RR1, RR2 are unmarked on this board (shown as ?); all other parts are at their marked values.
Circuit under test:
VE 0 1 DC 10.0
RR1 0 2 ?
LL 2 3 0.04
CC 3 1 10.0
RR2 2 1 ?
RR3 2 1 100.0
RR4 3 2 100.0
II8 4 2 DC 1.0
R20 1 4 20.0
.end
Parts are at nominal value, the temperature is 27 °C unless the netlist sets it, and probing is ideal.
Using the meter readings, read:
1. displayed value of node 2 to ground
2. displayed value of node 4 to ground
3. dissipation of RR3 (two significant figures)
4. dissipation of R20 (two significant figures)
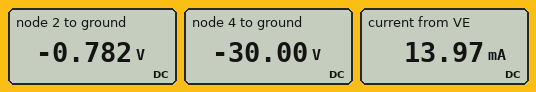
-0.782 V
-30.00 V
850 mW
20 W
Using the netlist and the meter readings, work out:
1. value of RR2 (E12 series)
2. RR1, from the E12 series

10 Ω
56 Ω
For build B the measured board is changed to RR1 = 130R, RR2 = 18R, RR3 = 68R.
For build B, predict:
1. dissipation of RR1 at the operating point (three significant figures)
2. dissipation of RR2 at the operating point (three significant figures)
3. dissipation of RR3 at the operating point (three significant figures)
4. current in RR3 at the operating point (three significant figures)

112 mW
10.6 W
2.81 W
203 mA
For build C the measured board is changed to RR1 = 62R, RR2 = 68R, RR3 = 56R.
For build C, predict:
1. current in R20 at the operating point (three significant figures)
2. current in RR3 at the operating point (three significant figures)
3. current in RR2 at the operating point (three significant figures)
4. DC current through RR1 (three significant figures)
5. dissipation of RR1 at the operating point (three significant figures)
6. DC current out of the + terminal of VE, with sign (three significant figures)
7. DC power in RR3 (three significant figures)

1.00 A
426 mA
351 mA
223 mA
3.09 W
-223 mA
10.2 W
